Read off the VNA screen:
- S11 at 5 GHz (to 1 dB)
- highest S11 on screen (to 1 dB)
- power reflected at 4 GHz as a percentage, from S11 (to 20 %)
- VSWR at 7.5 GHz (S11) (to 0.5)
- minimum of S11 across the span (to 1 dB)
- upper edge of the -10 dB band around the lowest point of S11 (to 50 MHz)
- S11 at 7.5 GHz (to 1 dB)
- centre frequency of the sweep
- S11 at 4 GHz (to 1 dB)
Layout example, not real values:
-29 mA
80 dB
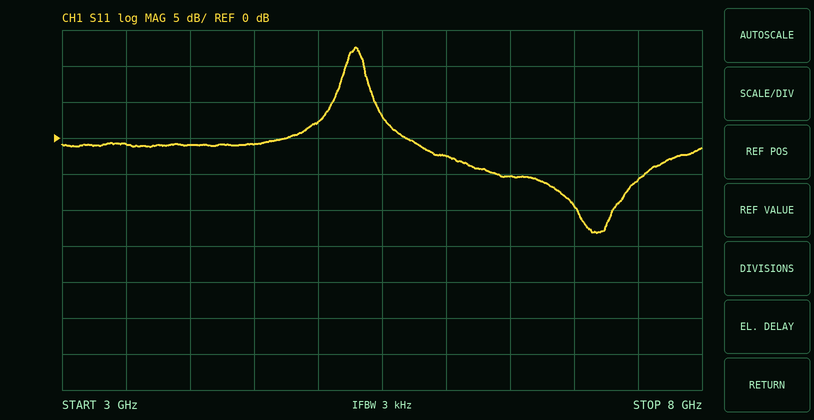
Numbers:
2 dB
13 dB
80 %
3.0
-13 dB
7.30 GHz
-6 dB
5.5 GHz
-1 dB
